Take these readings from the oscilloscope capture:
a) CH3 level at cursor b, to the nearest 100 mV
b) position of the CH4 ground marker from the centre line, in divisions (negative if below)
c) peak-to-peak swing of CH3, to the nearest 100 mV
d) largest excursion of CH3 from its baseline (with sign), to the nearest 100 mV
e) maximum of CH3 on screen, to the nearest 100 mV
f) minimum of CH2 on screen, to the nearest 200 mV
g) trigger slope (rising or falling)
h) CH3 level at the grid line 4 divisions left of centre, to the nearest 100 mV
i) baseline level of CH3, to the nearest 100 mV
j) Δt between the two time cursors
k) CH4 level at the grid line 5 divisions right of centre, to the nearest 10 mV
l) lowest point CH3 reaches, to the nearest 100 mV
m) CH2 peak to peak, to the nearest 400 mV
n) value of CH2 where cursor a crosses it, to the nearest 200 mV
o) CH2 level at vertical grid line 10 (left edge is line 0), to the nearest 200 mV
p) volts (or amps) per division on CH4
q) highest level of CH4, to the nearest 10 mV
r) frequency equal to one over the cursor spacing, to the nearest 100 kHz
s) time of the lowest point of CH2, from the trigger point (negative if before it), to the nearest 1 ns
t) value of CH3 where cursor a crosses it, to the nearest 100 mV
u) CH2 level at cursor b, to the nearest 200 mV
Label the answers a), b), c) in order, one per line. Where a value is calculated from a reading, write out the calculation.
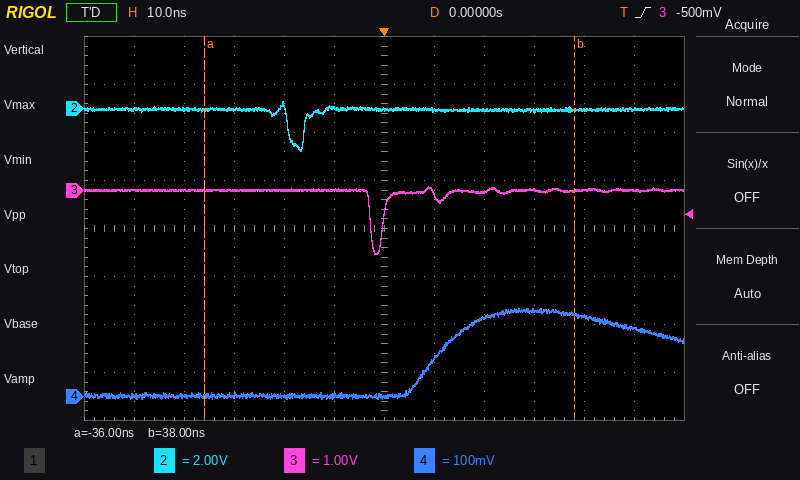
a) 0.0 V
b) -3.5 div
c) 100 mV − (-1.3 V) = 1.4 V
d) -1.3 V − (0.0 V) = -1.3 V
e) 100 mV
f) -1.8 V
g) rising
h) 0.0 V
i) 0.0 V
j) 38 ns − (-36 ns) = 74 ns
k) 140 mV
l) -1.3 V
m) 2.0 V
n) 0.0 V
o) 0.0 V
p) 100 mV
q) 180 mV
r) 1 / 74 ns ≈ 13.5 MHz
s) -17 ns
t) 0.0 V
u) 0.0 V
